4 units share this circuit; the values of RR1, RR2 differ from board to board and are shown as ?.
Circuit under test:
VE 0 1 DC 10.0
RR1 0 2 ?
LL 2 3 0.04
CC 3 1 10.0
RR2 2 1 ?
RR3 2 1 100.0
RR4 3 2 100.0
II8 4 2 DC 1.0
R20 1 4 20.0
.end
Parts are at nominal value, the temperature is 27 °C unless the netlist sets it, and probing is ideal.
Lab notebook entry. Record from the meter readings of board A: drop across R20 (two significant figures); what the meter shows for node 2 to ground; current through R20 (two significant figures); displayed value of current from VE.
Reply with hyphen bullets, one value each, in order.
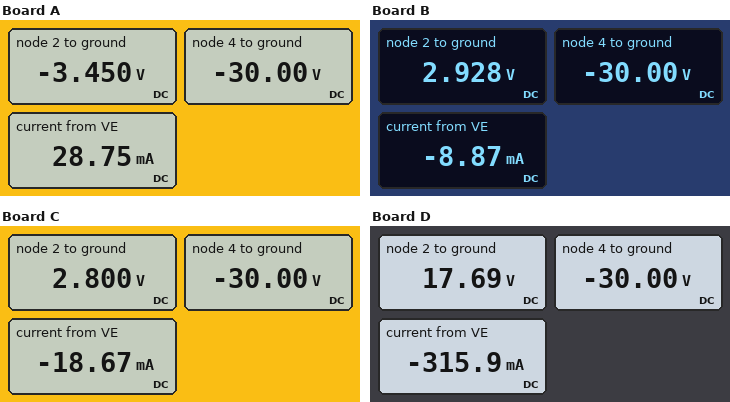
- 20 V
- -3.450 V
- 1.0 A
- 28.75 mA
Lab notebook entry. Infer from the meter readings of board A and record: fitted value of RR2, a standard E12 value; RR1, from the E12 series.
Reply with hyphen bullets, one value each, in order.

- 6.8 Ω
- 120 Ω
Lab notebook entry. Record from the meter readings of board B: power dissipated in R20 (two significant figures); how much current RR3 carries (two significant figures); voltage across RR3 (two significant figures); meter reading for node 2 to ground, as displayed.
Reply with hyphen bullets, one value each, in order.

- 20 W
- 130 mA
- 13 V
- 2.928 V
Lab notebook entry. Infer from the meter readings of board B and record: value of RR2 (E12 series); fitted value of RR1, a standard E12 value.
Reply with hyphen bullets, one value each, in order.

- 15 Ω
- 330 Ω
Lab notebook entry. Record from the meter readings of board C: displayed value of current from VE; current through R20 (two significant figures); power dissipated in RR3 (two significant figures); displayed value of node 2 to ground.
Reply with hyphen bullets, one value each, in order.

- -18.67 mA
- 1.0 A
- 1.6 W
- 2.800 V
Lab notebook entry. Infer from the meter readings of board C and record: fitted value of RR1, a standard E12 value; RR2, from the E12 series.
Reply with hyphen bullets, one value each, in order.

- 150 Ω
- 15 Ω
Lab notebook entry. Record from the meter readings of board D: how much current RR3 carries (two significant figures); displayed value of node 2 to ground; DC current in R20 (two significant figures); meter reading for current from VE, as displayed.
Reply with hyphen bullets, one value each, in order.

- 280 mA
- 17.69 V
- 1.0 A
- -315.9 mA
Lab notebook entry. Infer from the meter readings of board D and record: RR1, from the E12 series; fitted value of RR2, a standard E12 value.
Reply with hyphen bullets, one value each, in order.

- 56 Ω
- 68 Ω
